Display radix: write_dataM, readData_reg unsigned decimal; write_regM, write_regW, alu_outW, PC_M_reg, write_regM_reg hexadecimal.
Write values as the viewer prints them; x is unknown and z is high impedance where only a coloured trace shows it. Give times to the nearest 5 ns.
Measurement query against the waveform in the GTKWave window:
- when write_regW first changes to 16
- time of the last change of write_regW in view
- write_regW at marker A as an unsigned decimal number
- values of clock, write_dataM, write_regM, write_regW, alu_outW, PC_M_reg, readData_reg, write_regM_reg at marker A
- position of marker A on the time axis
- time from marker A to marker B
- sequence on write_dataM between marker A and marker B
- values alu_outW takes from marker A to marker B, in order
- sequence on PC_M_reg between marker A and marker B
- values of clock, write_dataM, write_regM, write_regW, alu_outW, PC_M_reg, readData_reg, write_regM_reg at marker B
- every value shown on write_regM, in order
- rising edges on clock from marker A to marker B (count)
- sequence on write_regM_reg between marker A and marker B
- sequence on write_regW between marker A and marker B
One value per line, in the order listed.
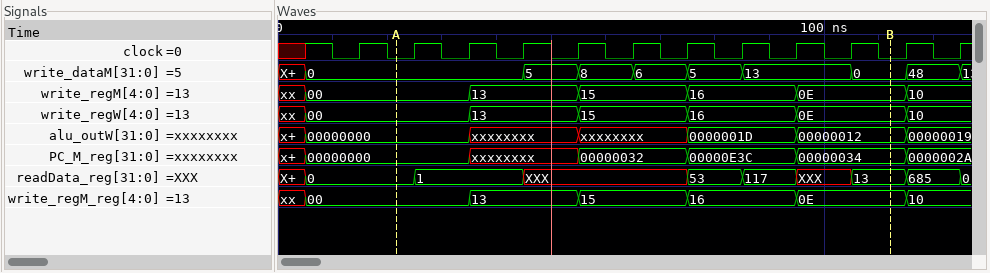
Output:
75 ns
115 ns
0
clock=0, write_dataM=0, write_regM=00, write_regW=00, alu_outW=00000000, PC_M_reg=00000000, readData_reg=0, write_regM_reg=00
20 ns
90 ns
0, 5, 8, 6, 5, 13, 0
00000000, xxxxxxxx, xxxxxxxx, 0000001D, 00000012
00000000, xxxxxxxx, 00000032, 00000E3C, 00000034
clock=0, write_dataM=0, write_regM=0E, write_regW=0E, alu_outW=00000012, PC_M_reg=00000034, readData_reg=13, write_regM_reg=0E
xx, 00, 13, 15, 16, 0E, 10
9
00, 13, 15, 16, 0E
00, 13, 15, 16, 0E
